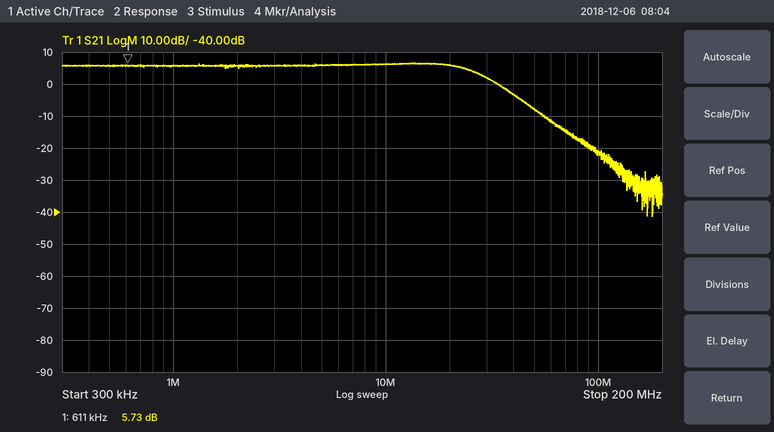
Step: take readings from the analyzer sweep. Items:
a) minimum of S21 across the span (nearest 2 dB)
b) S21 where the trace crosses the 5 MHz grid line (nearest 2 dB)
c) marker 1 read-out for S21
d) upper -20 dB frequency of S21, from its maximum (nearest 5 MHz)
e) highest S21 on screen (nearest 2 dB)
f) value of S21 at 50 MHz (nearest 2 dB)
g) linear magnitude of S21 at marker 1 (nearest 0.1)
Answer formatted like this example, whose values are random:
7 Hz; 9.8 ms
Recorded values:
-42 dB; 6 dB; 5.73 dB; 65 MHz; 6 dB; -8 dB; 1.9
